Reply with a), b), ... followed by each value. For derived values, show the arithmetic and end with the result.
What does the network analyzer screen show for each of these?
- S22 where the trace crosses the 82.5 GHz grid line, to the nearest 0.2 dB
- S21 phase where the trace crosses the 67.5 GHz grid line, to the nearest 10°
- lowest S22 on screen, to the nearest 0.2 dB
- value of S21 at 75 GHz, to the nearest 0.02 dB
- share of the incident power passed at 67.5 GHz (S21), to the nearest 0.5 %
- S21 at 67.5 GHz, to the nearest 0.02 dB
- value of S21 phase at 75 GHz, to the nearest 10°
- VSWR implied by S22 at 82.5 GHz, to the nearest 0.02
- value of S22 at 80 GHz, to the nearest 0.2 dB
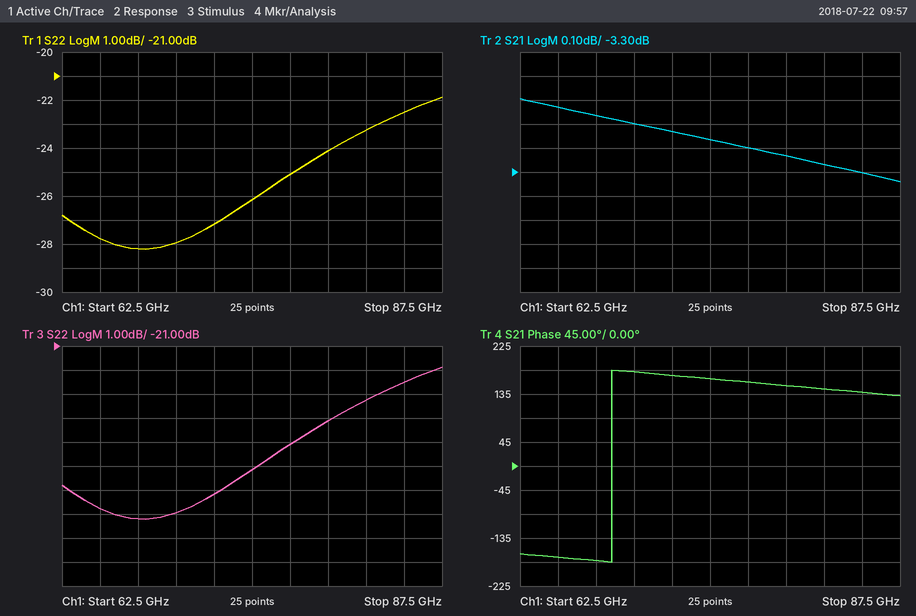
a) -23.2 dB
b) -180°
c) -28.2 dB
d) -3.16 dB
e) 10^(-3.06/10) ≈ 49.4 %, so 49.5 % to the nearest 0.5 %
f) -3.06 dB
g) 160°
h) |Γ| = 10^(-23.2/20) = 0.0692; VSWR = (1 + 0.0692)/(1 − 0.0692) ≈ 1.15, so 1.14 to the nearest 0.02
i) -24.2 dB
